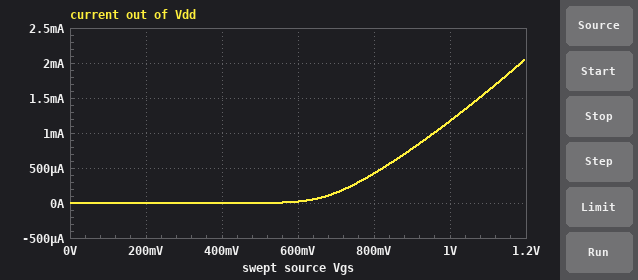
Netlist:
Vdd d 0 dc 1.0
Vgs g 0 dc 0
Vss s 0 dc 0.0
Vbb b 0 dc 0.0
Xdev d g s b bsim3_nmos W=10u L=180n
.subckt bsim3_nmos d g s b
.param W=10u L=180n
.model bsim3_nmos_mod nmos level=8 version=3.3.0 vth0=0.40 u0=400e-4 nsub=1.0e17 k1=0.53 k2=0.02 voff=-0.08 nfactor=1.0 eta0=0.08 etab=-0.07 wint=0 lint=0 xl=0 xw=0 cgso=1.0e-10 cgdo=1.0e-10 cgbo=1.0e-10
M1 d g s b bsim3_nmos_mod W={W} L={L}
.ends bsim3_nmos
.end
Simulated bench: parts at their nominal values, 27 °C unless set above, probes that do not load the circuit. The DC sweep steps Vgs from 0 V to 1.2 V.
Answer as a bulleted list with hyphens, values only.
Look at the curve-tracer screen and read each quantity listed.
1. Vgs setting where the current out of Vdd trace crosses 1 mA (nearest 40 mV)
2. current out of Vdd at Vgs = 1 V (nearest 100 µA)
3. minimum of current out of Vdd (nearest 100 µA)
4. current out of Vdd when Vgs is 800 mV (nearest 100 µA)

- 960 mV
- 1.2 mA
- 0 A
- 400 µA
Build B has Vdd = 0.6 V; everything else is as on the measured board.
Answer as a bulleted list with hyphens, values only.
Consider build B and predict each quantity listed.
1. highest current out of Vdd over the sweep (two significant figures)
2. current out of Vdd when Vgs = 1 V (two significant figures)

- 1.8 mA
- 1.0 mA
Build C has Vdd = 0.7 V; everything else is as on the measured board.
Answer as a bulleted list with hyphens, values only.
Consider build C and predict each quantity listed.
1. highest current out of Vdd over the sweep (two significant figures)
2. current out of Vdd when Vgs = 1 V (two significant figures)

- 1.9 mA
- 1.1 mA
